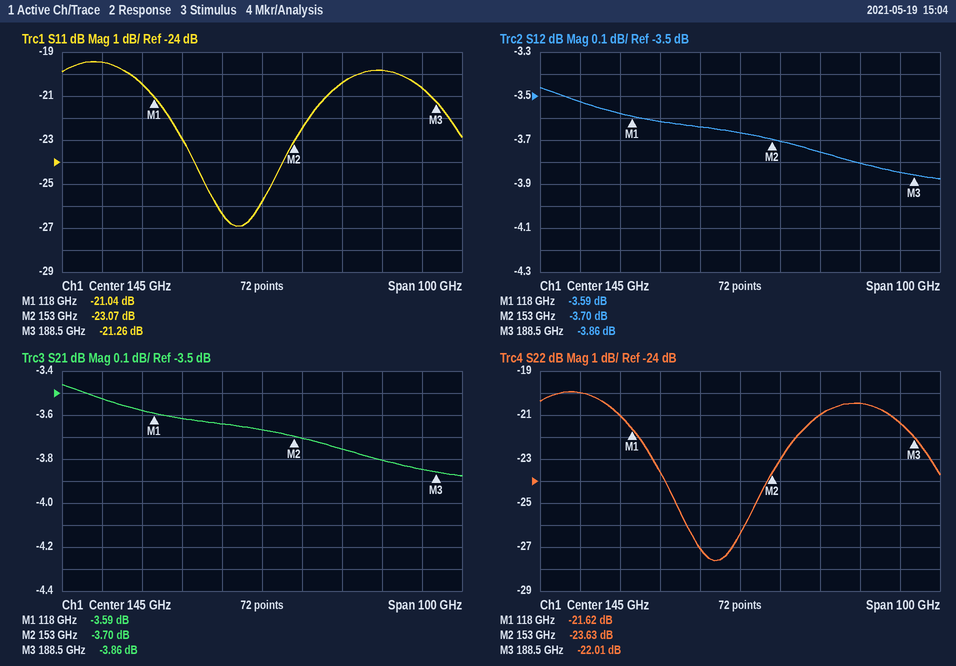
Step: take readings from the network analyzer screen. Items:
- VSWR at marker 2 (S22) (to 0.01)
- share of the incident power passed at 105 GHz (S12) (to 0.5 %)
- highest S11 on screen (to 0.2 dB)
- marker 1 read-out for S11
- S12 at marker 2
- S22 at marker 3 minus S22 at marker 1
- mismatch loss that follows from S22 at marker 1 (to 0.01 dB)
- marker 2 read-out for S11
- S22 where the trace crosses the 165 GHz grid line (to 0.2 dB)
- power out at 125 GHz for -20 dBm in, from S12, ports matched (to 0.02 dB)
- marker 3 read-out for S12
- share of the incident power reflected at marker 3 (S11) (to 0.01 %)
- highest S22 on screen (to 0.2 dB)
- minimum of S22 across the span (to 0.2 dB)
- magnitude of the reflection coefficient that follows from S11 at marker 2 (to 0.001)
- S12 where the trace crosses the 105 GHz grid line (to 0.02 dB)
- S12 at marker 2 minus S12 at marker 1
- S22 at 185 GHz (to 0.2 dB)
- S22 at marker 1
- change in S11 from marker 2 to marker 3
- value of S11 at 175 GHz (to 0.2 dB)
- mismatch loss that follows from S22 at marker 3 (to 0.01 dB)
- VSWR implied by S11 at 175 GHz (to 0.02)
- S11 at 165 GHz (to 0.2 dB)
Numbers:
1.14
44.5 %
-19.4 dB
-21.04 dB
-3.70 dB
-0.39 dB
0.03 dB
-23.07 dB
-21.0 dB
-23.62 dBm
-3.86 dB
0.75 %
-20.0 dB
-27.6 dB
0.070
-3.52 dB
-0.11 dB
-21.4 dB
-21.62 dB
1.81 dB
-19.8 dB
0.03 dB
1.22
-20.4 dB
